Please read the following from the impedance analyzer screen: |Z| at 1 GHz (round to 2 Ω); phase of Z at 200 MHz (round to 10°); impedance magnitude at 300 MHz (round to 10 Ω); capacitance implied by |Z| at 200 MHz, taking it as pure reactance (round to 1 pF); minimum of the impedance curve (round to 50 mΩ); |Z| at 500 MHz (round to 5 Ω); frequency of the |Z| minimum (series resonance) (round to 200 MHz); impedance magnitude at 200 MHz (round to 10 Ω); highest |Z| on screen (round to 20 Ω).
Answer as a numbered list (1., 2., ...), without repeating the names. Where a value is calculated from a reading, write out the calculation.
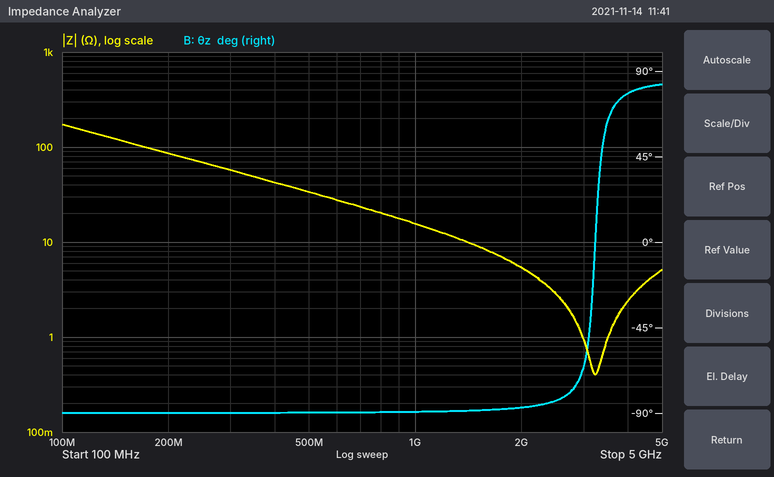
1. 16 Ω
2. -90°
3. 60 Ω
4. C = 1/(2π × 200 MHz × 90 Ω) ≈ 9 pF
5. 400 mΩ
6. 35 Ω
7. 3.2 GHz
8. 90 Ω
9. 180 Ω
